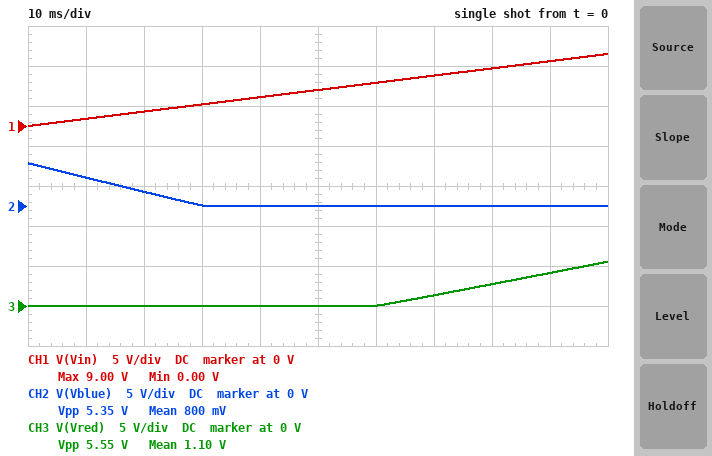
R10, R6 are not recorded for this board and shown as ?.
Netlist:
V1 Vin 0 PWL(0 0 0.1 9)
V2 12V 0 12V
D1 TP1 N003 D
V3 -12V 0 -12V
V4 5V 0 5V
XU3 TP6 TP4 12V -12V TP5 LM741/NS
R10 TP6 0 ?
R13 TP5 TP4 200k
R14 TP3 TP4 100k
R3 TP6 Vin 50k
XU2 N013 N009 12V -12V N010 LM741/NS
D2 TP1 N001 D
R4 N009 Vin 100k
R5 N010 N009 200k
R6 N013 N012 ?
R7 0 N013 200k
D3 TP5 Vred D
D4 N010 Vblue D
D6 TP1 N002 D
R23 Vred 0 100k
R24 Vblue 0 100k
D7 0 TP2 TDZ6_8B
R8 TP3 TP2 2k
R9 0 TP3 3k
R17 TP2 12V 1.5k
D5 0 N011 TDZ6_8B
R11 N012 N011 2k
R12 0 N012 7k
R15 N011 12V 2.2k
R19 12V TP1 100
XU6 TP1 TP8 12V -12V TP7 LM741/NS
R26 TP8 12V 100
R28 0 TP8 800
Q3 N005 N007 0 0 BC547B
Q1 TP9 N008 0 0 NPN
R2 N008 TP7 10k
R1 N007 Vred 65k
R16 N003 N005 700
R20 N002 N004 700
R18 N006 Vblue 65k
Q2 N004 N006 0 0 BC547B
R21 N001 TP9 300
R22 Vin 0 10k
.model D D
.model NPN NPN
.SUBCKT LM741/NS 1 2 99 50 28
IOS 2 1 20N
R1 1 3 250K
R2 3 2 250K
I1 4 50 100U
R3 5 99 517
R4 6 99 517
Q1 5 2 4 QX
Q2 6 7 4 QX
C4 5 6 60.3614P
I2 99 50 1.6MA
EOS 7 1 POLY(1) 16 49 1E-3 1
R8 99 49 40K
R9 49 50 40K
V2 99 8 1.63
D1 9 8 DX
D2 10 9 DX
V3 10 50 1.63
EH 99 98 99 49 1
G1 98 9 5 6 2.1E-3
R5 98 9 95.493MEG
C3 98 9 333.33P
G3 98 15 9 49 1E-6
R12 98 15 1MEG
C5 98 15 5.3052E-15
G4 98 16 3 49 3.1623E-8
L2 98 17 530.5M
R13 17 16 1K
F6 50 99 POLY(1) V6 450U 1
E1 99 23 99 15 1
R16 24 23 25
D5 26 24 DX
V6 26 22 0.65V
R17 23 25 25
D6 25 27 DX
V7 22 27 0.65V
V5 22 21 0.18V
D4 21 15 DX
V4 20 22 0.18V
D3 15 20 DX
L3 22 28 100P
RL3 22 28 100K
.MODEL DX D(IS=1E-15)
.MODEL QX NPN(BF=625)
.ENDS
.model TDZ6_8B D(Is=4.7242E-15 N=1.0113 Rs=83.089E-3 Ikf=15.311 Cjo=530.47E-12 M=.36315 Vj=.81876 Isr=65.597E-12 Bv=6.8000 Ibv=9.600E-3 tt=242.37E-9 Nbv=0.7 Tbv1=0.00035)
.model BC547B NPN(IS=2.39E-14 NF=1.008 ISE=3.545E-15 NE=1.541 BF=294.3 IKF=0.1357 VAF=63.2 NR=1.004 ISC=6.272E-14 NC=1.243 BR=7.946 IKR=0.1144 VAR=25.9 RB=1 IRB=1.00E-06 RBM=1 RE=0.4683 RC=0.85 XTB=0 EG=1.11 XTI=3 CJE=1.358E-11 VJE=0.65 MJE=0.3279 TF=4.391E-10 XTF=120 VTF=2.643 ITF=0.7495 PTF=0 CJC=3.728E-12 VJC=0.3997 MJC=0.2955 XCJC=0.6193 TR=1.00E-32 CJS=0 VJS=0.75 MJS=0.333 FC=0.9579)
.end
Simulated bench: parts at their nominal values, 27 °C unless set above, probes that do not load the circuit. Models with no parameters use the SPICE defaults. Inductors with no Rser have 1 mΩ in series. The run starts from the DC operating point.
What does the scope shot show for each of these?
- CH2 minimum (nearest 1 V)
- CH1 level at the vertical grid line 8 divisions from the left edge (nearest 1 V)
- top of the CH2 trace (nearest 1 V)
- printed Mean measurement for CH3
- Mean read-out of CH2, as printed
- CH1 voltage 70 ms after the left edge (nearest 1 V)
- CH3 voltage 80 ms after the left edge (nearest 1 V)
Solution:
0 V
7 V
5 V
1.10 V
800 mV
6 V
3 V
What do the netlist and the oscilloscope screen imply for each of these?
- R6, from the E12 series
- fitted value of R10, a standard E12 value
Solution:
330 kΩ
56 kΩ
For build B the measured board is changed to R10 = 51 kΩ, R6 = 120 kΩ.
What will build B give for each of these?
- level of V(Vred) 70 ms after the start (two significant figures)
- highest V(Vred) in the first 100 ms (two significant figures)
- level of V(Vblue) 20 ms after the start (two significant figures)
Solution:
910 mV
4.9 V
5.6 V
